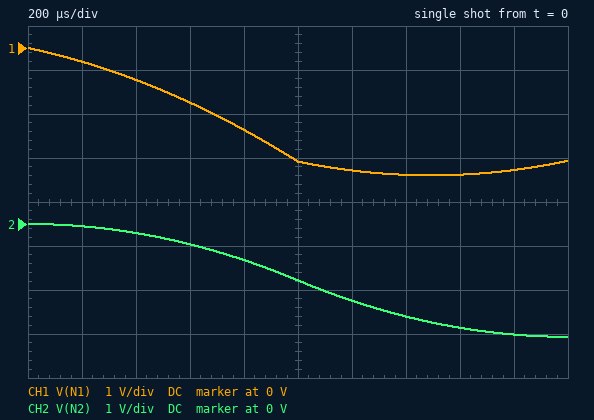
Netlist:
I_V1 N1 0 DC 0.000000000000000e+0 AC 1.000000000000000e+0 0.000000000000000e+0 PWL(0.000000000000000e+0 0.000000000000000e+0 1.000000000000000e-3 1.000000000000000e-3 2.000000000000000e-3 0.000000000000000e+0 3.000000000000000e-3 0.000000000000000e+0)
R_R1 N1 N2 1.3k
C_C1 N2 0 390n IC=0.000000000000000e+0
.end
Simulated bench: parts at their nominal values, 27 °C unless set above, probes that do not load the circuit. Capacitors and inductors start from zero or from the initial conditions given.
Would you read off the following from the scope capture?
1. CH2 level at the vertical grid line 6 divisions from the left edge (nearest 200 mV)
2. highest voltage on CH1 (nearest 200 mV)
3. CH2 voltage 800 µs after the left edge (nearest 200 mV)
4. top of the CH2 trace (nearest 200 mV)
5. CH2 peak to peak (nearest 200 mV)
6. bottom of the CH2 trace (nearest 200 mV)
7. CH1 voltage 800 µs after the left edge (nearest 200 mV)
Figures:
-1.8 V
0 V
-800 mV
0 V
2.6 V
-2.6 V
-1.8 V
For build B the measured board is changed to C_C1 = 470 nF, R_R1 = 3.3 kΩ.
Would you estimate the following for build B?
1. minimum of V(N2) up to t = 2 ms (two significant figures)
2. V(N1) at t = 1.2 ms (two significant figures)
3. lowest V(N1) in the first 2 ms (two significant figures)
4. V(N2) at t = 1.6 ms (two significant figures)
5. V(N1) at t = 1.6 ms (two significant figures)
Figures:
-2.1 V
-4.1 V
-4.4 V
-2.0 V
-3.3 V
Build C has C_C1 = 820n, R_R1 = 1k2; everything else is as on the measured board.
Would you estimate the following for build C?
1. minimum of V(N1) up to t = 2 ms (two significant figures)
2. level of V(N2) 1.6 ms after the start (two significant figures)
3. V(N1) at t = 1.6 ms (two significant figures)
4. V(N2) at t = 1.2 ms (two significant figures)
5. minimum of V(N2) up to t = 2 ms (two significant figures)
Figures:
-1.8 V
-1.1 V
-1.6 V
-830 mV
-1.2 V
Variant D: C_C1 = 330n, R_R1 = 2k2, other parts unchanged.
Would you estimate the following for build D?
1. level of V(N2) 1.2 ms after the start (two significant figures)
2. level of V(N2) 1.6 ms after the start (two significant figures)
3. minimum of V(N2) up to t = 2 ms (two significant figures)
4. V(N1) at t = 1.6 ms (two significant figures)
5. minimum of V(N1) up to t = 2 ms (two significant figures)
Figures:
-2.1 V
-2.8 V
-3.0 V
-3.7 V
-3.8 V
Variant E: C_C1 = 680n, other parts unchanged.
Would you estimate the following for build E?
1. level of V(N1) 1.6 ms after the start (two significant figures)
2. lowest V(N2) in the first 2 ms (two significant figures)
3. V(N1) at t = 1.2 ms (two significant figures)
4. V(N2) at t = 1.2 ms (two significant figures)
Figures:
-1.9 V
-1.5 V
-2.0 V
-1.0 V
